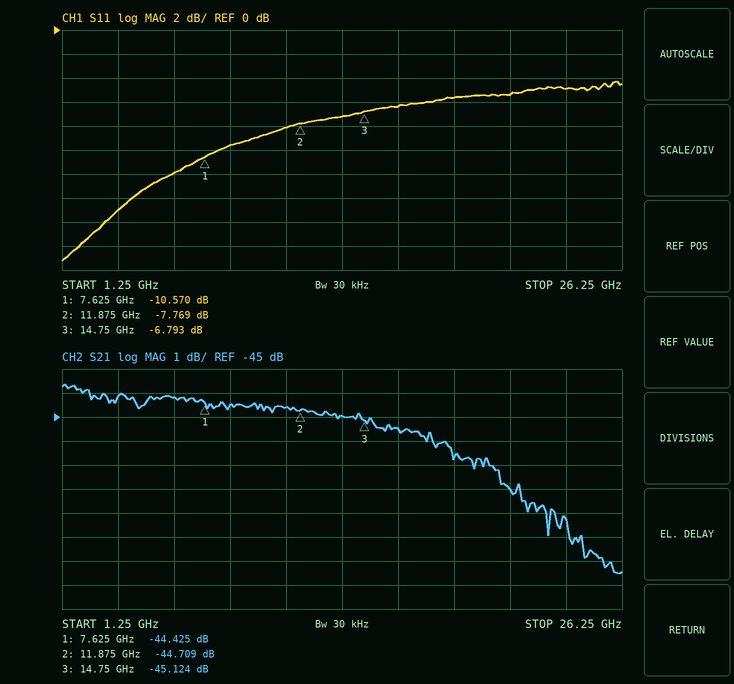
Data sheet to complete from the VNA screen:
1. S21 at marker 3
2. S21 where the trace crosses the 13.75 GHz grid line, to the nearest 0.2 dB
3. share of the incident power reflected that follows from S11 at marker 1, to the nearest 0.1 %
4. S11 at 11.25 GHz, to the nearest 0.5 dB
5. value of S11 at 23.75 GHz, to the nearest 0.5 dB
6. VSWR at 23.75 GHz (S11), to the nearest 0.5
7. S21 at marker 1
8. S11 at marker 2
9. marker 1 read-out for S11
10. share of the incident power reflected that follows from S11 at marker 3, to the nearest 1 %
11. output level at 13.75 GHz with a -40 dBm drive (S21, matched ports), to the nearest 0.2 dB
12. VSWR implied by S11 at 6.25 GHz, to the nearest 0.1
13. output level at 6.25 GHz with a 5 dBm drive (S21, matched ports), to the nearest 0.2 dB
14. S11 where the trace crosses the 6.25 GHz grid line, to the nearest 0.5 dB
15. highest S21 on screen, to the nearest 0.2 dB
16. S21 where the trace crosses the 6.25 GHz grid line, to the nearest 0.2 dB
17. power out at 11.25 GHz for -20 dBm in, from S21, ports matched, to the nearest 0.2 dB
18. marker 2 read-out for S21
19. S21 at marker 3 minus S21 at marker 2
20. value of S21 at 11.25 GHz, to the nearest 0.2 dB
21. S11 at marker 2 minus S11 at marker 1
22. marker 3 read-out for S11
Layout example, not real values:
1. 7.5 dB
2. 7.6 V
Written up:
1. -45.124 dB
2. -45.0 dB
3. 8.8 %
4. -8.0 dB
5. -5.0 dB
6. 3.5
7. -44.425 dB
8. -7.769 dB
9. -10.570 dB
10. 21 %
11. -85.0 dBm
12. 1.7
13. -39.2 dBm
14. -12.0 dB
15. -43.6 dB
16. -44.2 dB
17. -64.6 dBm
18. -44.709 dB
19. -0.415 dB
20. -44.6 dB
21. 2.801 dB
22. -6.793 dB
